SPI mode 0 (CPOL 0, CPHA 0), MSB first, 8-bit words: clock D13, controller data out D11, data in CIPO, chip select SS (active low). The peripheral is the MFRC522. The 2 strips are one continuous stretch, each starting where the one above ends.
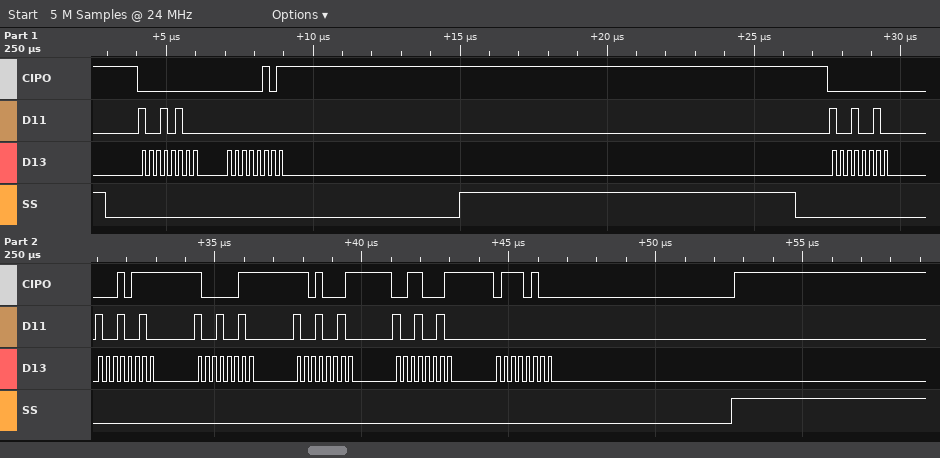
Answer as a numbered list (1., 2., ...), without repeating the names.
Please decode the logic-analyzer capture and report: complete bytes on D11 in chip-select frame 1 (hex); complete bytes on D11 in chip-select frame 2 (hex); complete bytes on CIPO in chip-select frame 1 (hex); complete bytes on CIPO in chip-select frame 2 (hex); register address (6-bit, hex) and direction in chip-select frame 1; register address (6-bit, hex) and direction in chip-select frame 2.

1. 94 00
2. 92 92 92 92 92 00
3. 00 05
4. 00 17 83 D1 31 74
5. 0x0A read
6. 0x09 read
